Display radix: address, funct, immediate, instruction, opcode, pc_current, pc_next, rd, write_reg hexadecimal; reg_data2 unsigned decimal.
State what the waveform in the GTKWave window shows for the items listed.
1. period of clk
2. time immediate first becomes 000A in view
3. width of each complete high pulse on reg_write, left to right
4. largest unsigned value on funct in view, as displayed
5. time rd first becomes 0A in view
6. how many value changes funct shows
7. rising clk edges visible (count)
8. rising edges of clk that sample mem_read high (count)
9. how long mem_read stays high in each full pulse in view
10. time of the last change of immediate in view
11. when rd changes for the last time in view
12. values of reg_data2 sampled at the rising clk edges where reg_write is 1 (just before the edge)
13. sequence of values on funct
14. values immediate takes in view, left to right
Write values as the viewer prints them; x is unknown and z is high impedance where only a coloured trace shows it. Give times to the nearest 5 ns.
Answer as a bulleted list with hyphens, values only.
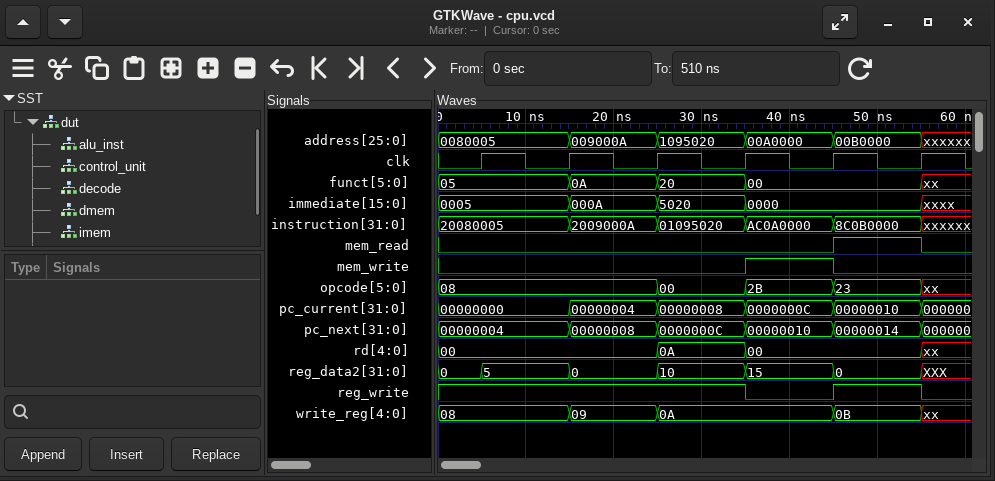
- 10 ns
- 15 ns
- 10 ns
- 20
- 25 ns
- 4
- 6
- 1
- 10 ns
- 55 ns
- 55 ns
- 0, 5, 0, 10, 0
- 05, 0A, 20, 00, xx
- 0005, 000A, 5020, 0000, xxxx
